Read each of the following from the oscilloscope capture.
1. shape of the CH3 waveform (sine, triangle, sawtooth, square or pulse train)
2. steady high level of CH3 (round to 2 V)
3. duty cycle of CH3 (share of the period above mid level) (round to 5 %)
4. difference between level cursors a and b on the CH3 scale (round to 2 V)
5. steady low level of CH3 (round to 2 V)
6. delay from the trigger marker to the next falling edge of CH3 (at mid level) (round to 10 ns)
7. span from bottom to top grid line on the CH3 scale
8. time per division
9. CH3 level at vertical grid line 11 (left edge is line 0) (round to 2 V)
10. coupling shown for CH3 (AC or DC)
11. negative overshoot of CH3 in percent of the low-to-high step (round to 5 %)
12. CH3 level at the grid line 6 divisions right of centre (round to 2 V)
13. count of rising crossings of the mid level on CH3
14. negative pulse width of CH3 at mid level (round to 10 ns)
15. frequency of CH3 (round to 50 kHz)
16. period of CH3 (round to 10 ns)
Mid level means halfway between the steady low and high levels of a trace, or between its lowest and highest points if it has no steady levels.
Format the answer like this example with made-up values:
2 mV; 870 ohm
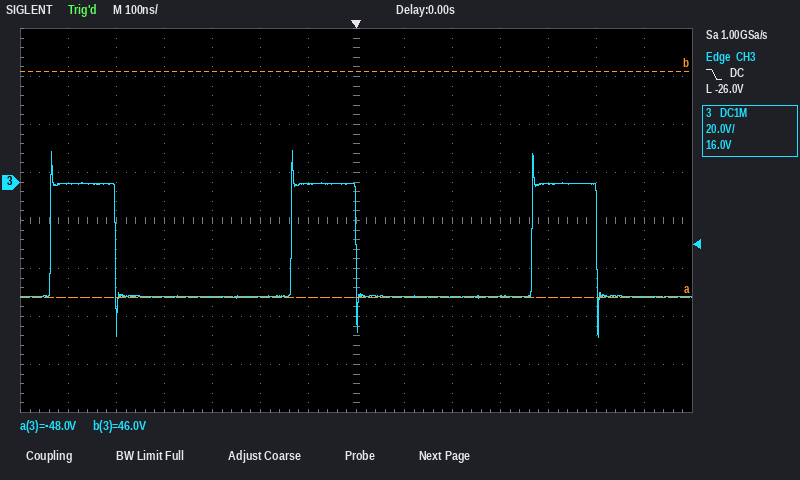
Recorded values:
pulse train; 0 V; 25 %; 94 V; -48 V; 500 ns; 160 V; 100 ns; 0 V; DC; 35 %; -48 V; 3; 370 ns; 2.00 MHz; 500 ns
